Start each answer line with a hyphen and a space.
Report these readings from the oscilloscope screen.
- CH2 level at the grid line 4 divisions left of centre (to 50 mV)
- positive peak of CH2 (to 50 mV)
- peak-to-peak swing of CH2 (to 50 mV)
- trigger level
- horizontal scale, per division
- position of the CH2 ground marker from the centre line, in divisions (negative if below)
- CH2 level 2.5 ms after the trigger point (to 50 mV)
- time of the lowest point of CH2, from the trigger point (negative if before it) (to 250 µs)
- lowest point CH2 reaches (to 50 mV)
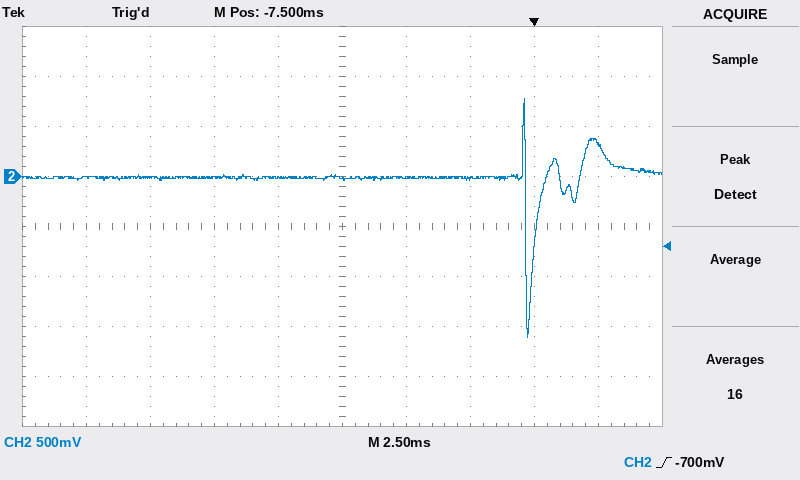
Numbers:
- 0 mV
- 800 mV
- 2.40 V
- -700 mV
- 2.5 ms
- +1.0 div
- 350 mV
- -250 µs
- -1.60 V
